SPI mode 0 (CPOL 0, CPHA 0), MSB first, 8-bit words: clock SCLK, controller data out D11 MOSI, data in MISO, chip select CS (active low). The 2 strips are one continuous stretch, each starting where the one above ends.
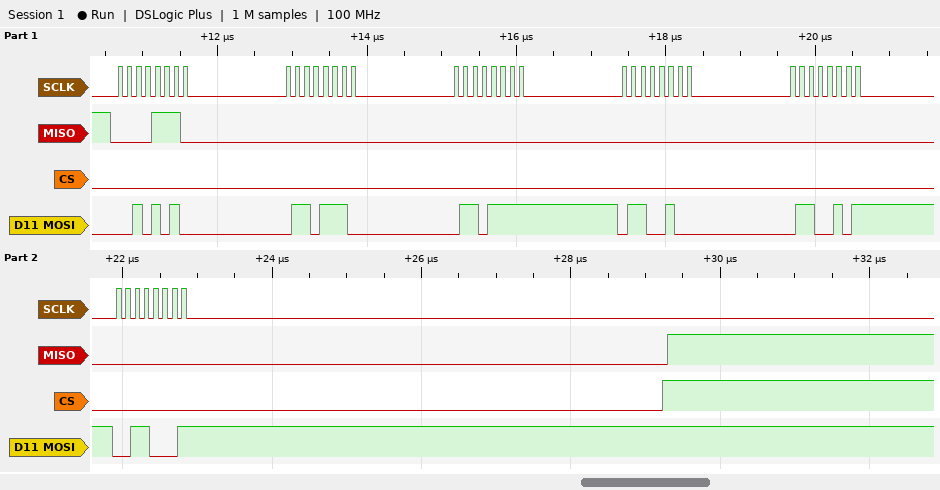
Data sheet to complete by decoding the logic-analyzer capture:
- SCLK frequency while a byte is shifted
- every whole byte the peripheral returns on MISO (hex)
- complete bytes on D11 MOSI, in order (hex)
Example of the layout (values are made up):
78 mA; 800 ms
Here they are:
8 MHz; 0E 00 00 00 00 00; 2A 6E 6F 64 65 31
